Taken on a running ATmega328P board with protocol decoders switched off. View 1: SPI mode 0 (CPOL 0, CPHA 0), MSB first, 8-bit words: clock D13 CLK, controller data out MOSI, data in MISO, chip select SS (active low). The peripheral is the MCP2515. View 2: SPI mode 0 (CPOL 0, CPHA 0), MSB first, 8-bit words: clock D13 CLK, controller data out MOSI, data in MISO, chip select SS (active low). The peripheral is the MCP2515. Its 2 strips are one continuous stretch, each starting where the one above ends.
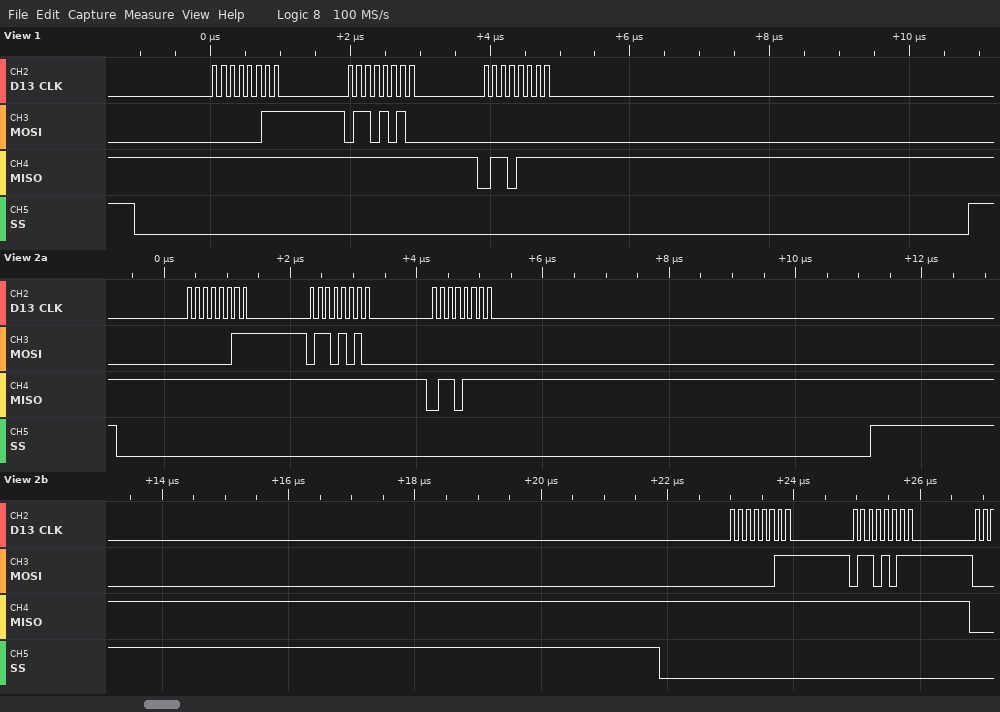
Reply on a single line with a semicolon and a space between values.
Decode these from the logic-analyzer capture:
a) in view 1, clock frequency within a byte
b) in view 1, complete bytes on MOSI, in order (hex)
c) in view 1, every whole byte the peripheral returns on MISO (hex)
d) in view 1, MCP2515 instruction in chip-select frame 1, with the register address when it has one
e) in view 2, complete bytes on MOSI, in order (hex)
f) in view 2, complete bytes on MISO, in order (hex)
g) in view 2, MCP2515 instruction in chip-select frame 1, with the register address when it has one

8 MHz; 03 6A 00; FF FF 6F; READ 0x6A; 03 6A 00 03 6B; FF FF 6F FF FF; READ 0x6A
